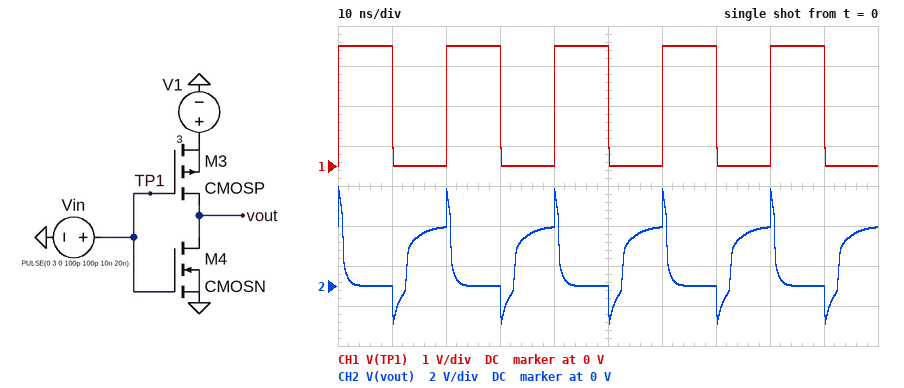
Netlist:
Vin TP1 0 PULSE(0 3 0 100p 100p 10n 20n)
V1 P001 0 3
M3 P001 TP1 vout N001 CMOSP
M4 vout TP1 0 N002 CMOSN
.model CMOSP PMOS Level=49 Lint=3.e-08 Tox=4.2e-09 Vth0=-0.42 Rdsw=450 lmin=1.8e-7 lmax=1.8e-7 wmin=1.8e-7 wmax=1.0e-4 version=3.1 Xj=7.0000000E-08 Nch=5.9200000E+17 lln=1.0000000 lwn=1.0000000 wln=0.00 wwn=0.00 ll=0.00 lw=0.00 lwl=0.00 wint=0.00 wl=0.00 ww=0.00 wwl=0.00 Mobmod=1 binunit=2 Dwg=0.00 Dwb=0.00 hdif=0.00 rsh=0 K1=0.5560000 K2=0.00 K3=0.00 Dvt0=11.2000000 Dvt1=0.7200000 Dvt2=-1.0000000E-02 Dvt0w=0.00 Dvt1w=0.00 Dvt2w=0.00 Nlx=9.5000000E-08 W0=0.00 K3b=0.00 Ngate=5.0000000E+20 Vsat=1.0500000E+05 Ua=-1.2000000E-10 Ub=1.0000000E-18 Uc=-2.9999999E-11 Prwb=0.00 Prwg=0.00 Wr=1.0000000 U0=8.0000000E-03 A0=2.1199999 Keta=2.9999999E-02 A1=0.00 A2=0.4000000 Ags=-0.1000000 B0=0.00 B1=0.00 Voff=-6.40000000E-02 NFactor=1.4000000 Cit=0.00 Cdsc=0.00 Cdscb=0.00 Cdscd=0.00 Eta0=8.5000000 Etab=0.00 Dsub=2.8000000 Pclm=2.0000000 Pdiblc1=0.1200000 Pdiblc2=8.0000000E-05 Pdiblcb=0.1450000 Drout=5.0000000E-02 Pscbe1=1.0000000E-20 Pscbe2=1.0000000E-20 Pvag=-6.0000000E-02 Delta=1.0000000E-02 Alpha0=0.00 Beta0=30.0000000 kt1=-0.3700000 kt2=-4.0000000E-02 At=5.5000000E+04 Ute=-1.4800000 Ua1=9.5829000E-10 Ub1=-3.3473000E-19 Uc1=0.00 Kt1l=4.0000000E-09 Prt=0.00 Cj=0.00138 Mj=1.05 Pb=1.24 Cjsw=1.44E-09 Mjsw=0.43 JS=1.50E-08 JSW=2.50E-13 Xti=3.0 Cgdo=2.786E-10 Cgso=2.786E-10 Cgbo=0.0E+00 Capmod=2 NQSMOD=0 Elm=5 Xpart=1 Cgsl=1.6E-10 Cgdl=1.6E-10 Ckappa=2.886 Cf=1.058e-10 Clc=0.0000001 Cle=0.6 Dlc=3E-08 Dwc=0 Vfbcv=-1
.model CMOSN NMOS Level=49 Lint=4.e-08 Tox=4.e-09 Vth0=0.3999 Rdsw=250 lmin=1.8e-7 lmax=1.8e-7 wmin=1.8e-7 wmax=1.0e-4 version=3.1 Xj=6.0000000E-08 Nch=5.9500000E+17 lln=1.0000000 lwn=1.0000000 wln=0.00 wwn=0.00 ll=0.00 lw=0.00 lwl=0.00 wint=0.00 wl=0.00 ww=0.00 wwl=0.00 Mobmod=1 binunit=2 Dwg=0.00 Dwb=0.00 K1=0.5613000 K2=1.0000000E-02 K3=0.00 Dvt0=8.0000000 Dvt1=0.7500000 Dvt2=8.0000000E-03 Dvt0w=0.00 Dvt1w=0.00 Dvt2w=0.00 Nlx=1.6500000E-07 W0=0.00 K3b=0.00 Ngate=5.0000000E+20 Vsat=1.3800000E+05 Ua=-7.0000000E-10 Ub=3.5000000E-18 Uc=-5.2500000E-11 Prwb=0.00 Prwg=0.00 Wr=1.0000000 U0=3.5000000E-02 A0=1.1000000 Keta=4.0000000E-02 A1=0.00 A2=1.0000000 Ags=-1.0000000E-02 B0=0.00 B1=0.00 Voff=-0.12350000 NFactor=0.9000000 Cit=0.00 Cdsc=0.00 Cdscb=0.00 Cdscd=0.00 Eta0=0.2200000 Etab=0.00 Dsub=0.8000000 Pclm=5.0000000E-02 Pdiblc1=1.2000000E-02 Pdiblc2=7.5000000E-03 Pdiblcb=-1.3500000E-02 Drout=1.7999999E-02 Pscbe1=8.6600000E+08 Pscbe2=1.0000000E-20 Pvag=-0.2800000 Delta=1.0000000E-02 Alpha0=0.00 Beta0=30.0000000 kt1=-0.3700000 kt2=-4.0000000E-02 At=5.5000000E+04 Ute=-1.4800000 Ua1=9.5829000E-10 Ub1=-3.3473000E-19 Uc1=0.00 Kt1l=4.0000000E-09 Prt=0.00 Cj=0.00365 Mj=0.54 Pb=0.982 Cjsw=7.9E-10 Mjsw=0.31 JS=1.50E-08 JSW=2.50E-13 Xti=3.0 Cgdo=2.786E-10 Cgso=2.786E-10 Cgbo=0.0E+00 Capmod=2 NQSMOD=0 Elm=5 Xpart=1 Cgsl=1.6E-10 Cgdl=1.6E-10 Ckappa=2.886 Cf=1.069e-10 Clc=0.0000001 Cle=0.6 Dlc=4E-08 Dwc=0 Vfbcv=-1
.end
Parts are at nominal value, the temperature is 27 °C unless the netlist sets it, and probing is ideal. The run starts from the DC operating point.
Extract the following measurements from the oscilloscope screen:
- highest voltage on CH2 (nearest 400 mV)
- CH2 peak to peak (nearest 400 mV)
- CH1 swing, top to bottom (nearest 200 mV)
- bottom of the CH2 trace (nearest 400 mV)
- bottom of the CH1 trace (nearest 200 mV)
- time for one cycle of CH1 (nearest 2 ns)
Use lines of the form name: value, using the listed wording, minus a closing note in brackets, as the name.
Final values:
highest voltage on CH2: 4.8 V
CH2 peak to peak: 6.8 V
CH1 swing, top to bottom: 3.0 V
bottom of the CH2 trace: -2.0 V
bottom of the CH1 trace: 0 V
time for one cycle of CH1: 20 ns
